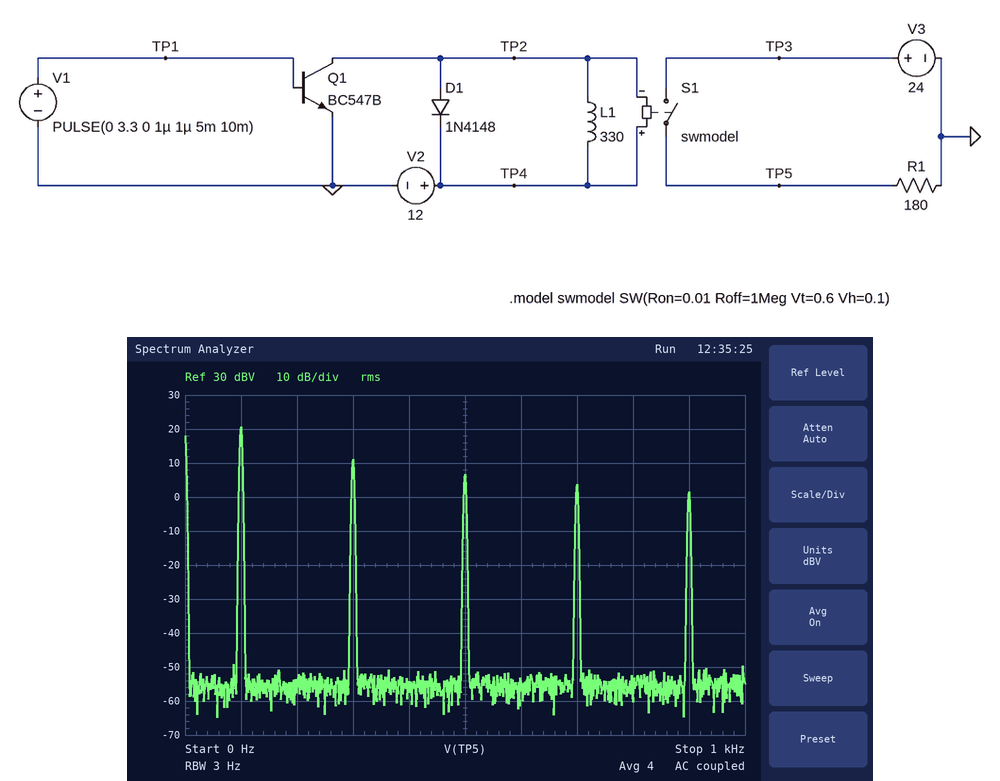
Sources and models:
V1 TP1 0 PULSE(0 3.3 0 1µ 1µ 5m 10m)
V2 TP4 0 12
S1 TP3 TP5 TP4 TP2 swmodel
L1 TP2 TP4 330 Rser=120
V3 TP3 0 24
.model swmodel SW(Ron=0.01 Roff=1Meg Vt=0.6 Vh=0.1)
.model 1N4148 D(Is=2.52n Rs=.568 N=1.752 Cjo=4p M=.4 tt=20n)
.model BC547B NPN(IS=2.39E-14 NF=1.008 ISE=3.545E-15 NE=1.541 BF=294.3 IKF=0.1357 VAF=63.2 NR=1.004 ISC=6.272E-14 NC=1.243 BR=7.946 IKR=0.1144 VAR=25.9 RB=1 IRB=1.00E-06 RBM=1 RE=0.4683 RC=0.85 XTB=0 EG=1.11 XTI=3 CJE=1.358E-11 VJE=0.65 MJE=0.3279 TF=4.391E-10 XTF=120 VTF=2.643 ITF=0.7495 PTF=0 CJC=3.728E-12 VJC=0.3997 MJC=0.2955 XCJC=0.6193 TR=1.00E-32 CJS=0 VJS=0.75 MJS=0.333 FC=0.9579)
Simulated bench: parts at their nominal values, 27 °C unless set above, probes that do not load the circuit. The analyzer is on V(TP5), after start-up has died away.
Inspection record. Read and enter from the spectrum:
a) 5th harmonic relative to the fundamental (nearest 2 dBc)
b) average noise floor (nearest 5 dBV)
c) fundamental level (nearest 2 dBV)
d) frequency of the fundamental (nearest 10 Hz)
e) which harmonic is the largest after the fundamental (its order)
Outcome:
-14 dBc
-55 dBV
20 dBV
100 Hz
3
